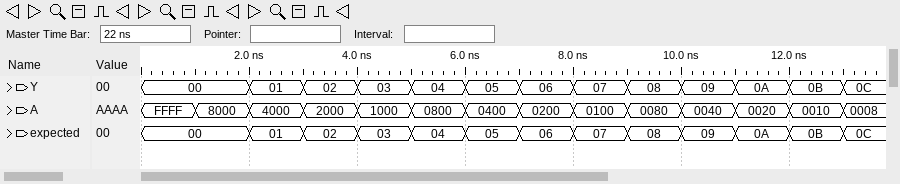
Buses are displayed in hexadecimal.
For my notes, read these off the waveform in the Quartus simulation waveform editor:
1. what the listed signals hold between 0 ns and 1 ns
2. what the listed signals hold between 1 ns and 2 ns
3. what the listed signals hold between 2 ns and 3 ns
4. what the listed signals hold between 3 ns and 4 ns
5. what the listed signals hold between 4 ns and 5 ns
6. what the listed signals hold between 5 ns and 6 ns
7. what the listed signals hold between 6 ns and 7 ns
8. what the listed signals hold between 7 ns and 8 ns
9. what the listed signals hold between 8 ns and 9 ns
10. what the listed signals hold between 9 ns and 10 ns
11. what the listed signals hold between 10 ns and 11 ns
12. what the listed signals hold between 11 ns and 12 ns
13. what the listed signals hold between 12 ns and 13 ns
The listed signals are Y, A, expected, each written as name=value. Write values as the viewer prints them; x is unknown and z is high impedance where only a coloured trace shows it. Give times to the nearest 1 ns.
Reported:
Y=00, A=FFFF, expected=00
Y=00, A=8000, expected=00
Y=01, A=4000, expected=01
Y=02, A=2000, expected=02
Y=03, A=1000, expected=03
Y=04, A=0800, expected=04
Y=05, A=0400, expected=05
Y=06, A=0200, expected=06
Y=07, A=0100, expected=07
Y=08, A=0080, expected=08
Y=09, A=0040, expected=09
Y=0A, A=0020, expected=0A
Y=0B, A=0010, expected=0B
